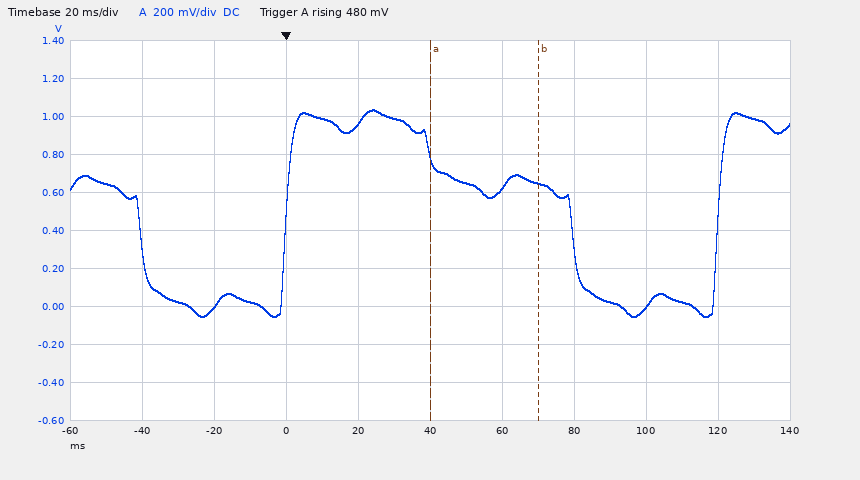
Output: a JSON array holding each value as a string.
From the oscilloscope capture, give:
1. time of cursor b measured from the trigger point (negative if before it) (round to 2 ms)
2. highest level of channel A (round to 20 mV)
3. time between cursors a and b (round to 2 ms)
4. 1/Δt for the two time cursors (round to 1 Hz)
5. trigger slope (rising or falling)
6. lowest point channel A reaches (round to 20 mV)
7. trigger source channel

["+70 ms", "1.04 V", "30 ms", "33 Hz", "rising", "-60 mV", "channel A"]
